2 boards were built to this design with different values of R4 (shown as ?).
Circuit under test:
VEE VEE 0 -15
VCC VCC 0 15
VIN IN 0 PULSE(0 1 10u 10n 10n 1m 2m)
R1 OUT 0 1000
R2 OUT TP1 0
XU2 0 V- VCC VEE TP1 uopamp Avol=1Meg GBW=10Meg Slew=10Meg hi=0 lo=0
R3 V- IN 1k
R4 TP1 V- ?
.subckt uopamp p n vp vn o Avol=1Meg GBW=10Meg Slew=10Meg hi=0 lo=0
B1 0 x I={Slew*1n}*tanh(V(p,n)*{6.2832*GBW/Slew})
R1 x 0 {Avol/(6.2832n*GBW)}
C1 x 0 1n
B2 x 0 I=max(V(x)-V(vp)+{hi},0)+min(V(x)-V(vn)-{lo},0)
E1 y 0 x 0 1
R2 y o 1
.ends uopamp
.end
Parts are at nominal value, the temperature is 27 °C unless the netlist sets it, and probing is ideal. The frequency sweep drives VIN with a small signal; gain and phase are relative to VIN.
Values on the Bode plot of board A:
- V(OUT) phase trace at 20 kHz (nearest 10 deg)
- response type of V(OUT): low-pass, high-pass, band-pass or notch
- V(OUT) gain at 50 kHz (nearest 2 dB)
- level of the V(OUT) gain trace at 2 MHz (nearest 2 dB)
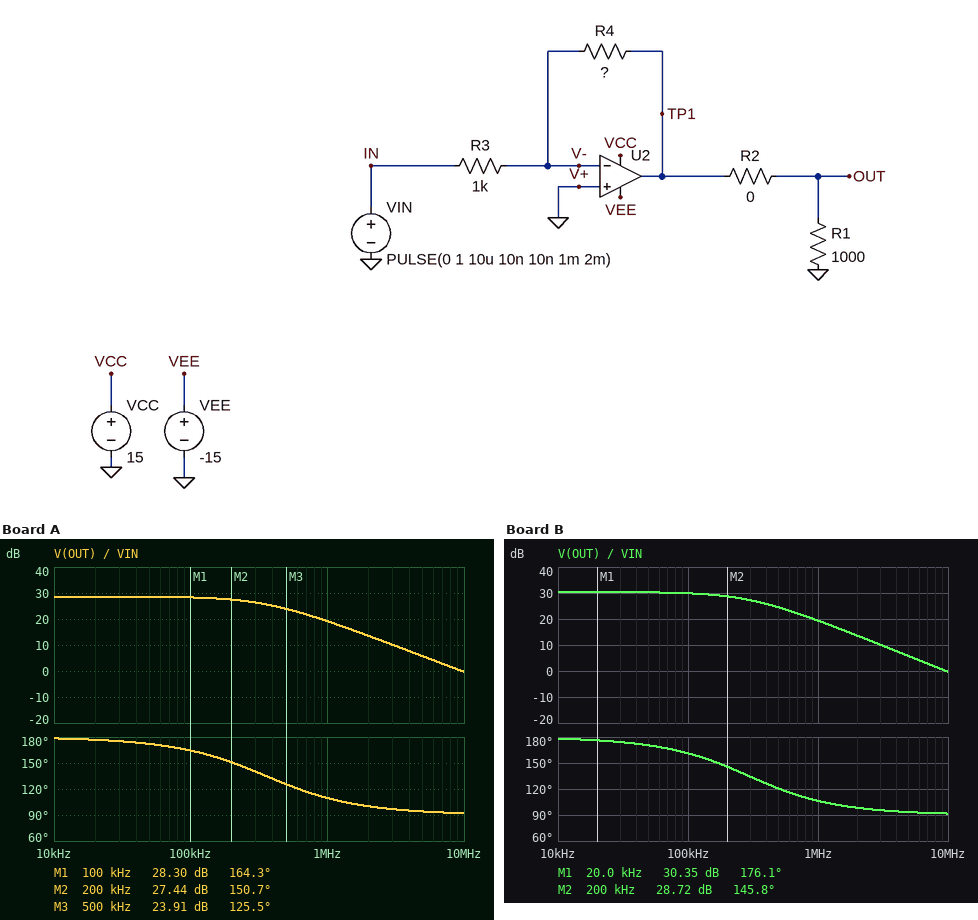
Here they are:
180 deg
low-pass
28 dB
14 dB
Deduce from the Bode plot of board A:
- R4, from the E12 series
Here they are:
27 kΩ
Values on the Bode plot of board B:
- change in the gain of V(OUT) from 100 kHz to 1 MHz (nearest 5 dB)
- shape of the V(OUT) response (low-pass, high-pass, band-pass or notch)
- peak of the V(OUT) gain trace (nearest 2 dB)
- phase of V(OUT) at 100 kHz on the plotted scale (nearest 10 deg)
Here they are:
-10 dB
low-pass
30 dB
160 deg
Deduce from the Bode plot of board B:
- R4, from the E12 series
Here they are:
33 kΩ
